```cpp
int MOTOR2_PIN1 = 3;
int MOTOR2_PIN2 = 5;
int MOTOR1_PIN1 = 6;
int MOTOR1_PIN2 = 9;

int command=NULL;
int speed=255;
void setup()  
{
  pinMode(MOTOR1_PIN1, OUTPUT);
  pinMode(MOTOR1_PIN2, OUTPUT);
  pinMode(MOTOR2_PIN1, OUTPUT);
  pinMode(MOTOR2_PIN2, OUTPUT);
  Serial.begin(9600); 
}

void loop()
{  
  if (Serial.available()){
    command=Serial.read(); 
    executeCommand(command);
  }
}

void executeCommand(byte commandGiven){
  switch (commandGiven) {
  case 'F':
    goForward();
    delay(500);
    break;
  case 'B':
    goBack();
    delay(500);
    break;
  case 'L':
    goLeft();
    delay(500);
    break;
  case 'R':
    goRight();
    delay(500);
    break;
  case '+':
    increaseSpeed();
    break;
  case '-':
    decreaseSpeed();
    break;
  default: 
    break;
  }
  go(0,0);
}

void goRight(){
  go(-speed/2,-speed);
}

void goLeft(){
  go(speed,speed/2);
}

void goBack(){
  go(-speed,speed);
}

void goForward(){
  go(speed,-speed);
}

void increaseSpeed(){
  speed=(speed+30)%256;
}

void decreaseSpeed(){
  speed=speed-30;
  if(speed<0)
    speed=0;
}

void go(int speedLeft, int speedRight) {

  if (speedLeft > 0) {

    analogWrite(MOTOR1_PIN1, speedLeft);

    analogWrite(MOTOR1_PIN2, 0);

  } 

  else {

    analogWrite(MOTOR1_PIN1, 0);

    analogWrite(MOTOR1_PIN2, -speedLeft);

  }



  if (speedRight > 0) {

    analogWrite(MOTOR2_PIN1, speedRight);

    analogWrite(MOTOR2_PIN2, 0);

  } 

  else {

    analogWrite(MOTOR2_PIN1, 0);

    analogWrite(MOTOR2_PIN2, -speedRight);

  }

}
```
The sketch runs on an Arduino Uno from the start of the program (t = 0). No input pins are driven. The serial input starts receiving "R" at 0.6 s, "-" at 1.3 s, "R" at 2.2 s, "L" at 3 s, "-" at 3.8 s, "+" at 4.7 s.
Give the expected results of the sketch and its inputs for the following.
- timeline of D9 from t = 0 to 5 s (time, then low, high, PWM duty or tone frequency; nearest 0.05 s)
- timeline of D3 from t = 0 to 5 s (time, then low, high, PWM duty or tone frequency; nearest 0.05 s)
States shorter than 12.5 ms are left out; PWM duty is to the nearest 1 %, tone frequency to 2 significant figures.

0 s low; 0.6 s PWM 50 %; 1.1 s low; 2.2 s PWM 44 %; 2.7 s low
0 s low; 3 s PWM 44 %; 3.5 s low
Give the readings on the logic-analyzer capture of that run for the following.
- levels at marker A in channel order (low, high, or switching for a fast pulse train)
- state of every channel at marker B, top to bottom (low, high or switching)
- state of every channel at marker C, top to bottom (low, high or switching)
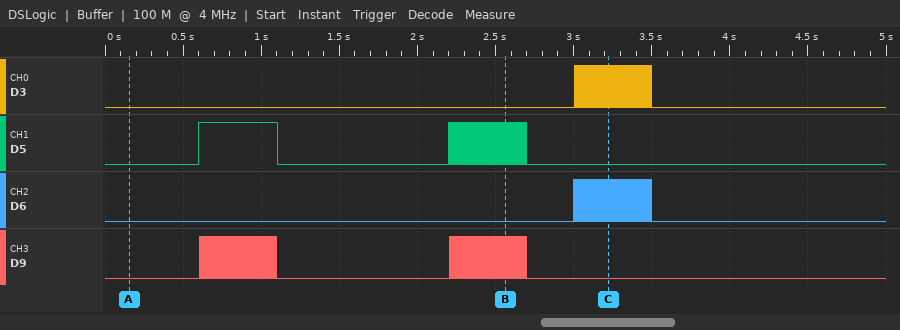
D3 low, D5 low, D6 low, D9 low
D3 low, D5 switching, D6 low, D9 switching
D3 switching, D5 low, D6 switching, D9 low
